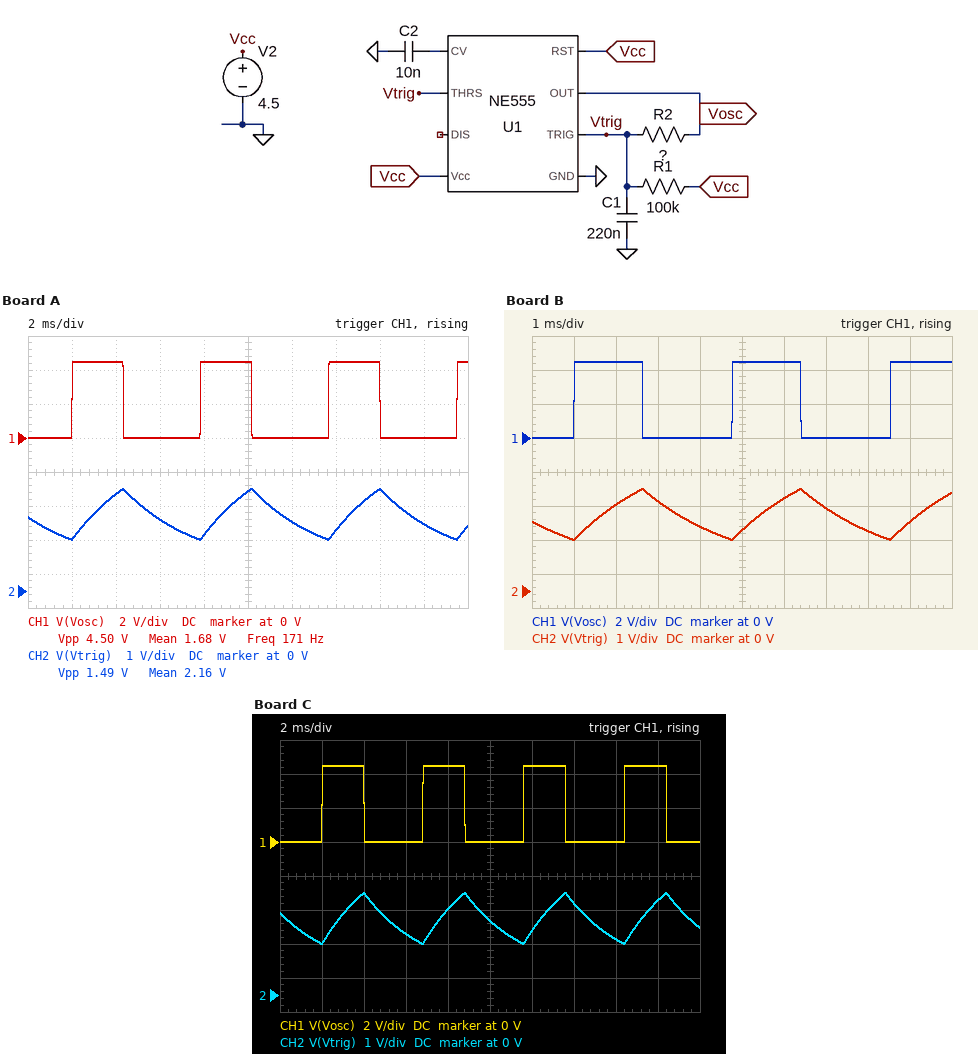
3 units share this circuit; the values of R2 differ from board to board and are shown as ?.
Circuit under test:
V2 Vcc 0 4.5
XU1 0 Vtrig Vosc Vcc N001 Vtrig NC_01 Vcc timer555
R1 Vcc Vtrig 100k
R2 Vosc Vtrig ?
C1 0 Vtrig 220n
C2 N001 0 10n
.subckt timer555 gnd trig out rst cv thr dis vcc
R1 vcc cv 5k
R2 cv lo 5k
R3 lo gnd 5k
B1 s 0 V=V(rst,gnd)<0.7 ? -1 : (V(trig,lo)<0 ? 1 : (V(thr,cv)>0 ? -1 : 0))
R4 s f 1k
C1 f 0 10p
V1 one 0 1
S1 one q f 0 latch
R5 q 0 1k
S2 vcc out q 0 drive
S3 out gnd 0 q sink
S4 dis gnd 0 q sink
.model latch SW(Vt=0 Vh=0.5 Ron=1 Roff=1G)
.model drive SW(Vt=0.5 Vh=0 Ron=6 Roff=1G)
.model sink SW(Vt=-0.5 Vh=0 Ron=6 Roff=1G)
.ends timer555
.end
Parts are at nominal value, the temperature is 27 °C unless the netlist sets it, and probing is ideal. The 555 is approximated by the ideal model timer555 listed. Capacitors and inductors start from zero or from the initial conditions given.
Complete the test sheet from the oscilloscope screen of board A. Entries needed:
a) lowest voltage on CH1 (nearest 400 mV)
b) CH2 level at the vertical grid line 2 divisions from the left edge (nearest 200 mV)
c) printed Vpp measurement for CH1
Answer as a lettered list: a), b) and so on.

a) 0 V
b) 2.8 V
c) 4.50 V
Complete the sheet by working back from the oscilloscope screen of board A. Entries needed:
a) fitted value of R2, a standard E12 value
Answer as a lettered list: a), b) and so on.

a) 18 kΩ
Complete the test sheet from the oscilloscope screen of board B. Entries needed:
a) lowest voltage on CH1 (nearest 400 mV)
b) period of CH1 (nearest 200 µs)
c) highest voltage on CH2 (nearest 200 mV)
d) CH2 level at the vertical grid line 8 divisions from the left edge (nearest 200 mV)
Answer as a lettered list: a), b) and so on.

a) 0 V
b) 3.8 ms
c) 3.0 V
d) 1.8 V
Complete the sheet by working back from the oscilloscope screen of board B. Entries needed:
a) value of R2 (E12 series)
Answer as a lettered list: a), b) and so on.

a) 12 kΩ
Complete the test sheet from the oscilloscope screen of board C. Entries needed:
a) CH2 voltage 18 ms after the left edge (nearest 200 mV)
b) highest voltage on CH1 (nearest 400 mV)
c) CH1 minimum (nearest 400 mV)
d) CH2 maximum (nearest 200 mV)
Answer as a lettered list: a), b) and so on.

a) 2.8 V
b) 4.4 V
c) 0 V
d) 3.0 V
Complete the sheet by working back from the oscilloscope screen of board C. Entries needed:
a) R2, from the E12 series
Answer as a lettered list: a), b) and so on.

a) 15 kΩ
